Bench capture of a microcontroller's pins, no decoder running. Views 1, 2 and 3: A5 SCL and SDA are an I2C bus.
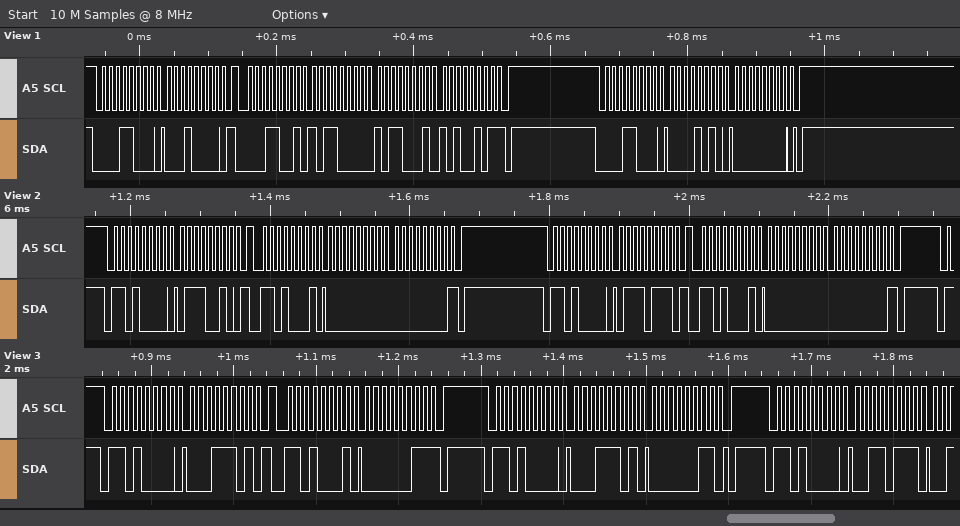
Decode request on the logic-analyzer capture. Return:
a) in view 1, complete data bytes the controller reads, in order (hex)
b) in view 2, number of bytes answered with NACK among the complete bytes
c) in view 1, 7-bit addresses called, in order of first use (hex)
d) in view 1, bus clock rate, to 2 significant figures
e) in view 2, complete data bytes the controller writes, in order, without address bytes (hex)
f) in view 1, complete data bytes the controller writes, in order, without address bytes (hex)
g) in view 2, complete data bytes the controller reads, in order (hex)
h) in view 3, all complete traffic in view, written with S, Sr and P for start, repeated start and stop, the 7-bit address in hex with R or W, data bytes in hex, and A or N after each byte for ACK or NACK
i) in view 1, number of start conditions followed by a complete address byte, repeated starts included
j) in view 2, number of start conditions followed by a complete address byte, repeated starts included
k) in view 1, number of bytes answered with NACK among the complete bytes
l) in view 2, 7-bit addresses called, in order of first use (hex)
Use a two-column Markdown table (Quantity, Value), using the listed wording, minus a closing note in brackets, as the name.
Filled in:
| Quantity | Value |
|---|---|
| in view 1, complete data bytes the controller reads, in order | B0 B1 A5 |
| in view 2, number of bytes answered with NACK among the complete bytes | 2 |
| in view 1, 7-bit addresses called, in order of first use | 0x0C |
| in view 1, bus clock rate, to 2 significant figures | 100 kHz |
| in view 2, complete data bytes the controller writes, in order, without address bytes | 72 77 |
| in view 1, complete data bytes the controller writes, in order, without address bytes | 10 0A 00 |
| in view 2, complete data bytes the controller reads, in order | 00 00 00 00 |
| in view 3, all complete traffic in view, written with S, Sr and P for start, repeated start and stop, the 7-bit address in hex with R or W, data bytes in hex, and A or N after each byte for ACK or NACK | S 68W A 1D A Sr 68R A 03 N P S 68W A 1D A 03 A P S 68W A 37 A |
| in view 1, number of start conditions followed by a complete address byte, repeated starts included | 3 |
| in view 2, number of start conditions followed by a complete address byte, repeated starts included | 4 |
| in view 1, number of bytes answered with NACK among the complete bytes | 1 |
| in view 2, 7-bit addresses called, in order of first use | 0x68 |
